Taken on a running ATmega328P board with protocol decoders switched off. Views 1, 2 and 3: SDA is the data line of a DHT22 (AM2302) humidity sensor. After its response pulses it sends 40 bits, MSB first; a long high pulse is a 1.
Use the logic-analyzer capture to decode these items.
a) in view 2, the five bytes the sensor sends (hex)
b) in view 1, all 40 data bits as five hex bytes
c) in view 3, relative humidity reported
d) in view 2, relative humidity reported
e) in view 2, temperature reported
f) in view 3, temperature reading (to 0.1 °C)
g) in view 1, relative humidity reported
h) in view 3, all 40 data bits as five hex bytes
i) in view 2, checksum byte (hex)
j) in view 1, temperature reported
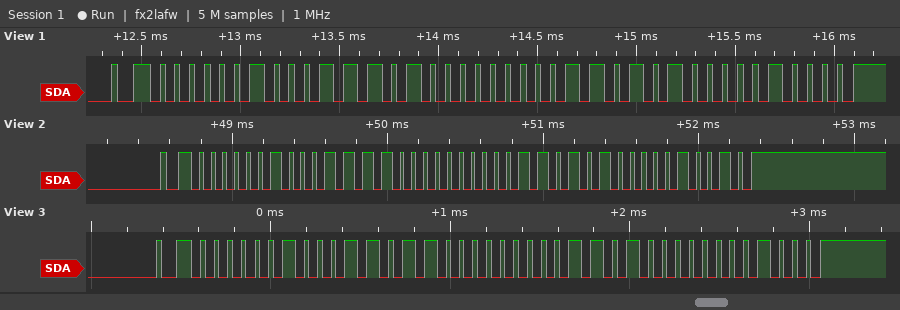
02 3C 00 D4 12
02 3A 00 D4 10
56.6 %
57.2 %
21.2 °C
20.8 °C
57.0 %
02 36 00 D0 08
0x12
21.2 °C
